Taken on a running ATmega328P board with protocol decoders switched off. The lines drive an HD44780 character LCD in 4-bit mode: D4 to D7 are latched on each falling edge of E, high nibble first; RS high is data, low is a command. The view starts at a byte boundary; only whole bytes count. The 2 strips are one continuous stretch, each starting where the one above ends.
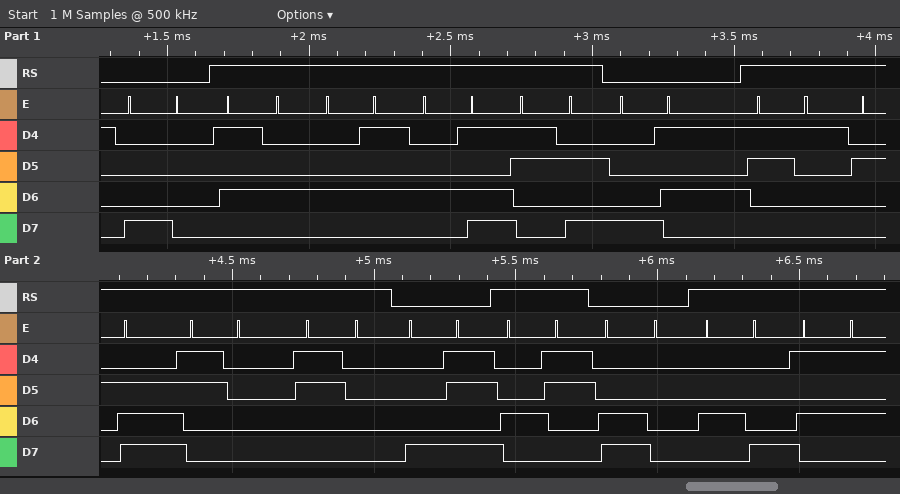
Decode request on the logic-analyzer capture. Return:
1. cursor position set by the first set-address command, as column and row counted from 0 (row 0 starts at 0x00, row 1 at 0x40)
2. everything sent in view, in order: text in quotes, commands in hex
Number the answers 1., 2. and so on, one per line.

1. column 0, row 0
2. 0x80 "TEM:" 0x85 "1.00" 0x8B "C" 0xC0 "HU"
